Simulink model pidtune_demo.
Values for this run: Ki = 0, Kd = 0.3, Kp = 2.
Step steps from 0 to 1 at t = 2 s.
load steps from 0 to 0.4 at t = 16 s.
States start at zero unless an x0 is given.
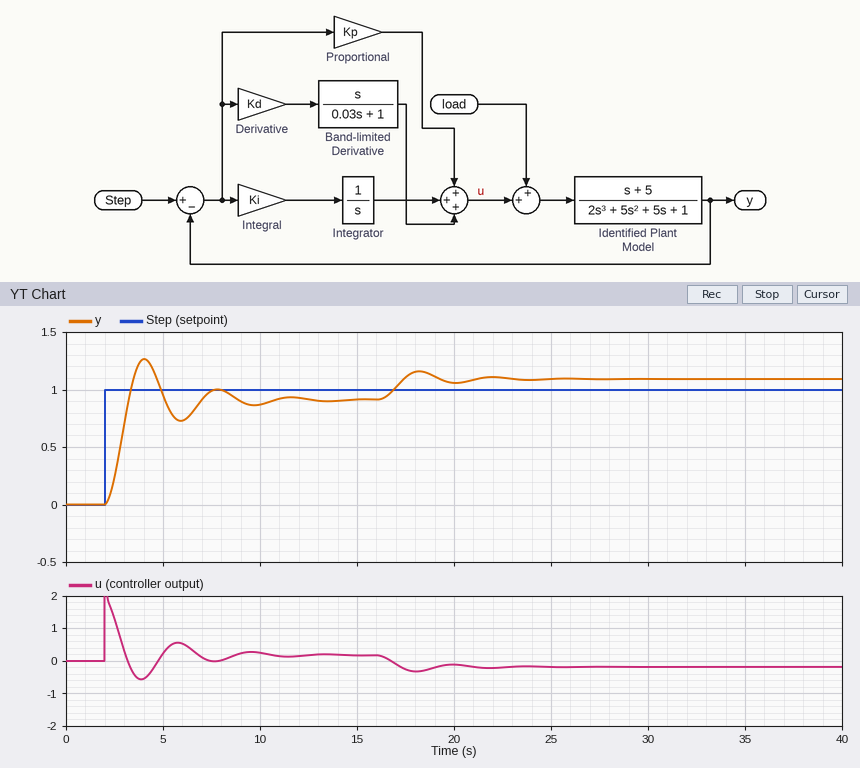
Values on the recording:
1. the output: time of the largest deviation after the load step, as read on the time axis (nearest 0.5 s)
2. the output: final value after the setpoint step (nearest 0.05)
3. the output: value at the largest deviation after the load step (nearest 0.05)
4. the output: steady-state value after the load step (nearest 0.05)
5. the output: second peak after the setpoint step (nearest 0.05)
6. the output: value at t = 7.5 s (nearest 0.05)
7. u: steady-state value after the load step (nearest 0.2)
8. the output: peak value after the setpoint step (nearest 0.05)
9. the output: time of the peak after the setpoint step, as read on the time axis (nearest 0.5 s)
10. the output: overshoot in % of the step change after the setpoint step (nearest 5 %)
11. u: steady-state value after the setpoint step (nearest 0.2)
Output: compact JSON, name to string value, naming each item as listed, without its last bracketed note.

{"the output: time of the largest deviation after the load step, as read on the time axis": "18.0 s", "the output: final value after the setpoint step": "0.90", "the output: value at the largest deviation after the load step": "1.15", "the output: steady-state value after the load step": "1.10", "the output: second peak after the setpoint step": "1.00", "the output: value at t = 7.5 s": "1.00", "u: steady-state value after the load step": "-0.2", "the output: peak value after the setpoint step": "1.25", "the output: time of the peak after the setpoint step, as read on the time axis": "4.0 s", "the output: overshoot in % of the step change after the setpoint step": "40 %", "u: steady-state value after the setpoint step": "0.2"}
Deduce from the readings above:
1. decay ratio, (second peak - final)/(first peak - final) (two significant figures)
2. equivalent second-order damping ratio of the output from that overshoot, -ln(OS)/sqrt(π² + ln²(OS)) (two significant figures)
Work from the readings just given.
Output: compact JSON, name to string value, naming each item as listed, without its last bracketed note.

{"decay ratio, (second peak - final)/(first peak - final)": "0.29", "equivalent second-order damping ratio of the output from that overshoot, -ln(OS)/sqrt(π² + ln²(OS))": "0.28"}
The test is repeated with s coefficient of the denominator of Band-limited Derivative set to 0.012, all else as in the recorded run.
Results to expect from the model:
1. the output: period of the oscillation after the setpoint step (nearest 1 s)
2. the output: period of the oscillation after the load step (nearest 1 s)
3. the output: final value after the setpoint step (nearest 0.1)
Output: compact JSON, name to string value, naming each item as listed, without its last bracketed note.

{"the output: period of the oscillation after the setpoint step": "4 s", "the output: period of the oscillation after the load step": "4 s", "the output: final value after the setpoint step": "0.9"}
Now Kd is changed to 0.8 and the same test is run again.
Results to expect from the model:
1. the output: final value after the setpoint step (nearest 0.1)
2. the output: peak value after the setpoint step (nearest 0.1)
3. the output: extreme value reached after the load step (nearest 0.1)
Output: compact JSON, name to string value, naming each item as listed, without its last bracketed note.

{"the output: final value after the setpoint step": "0.9", "the output: peak value after the setpoint step": "1.1", "the output: extreme value reached after the load step": "1.1"}
